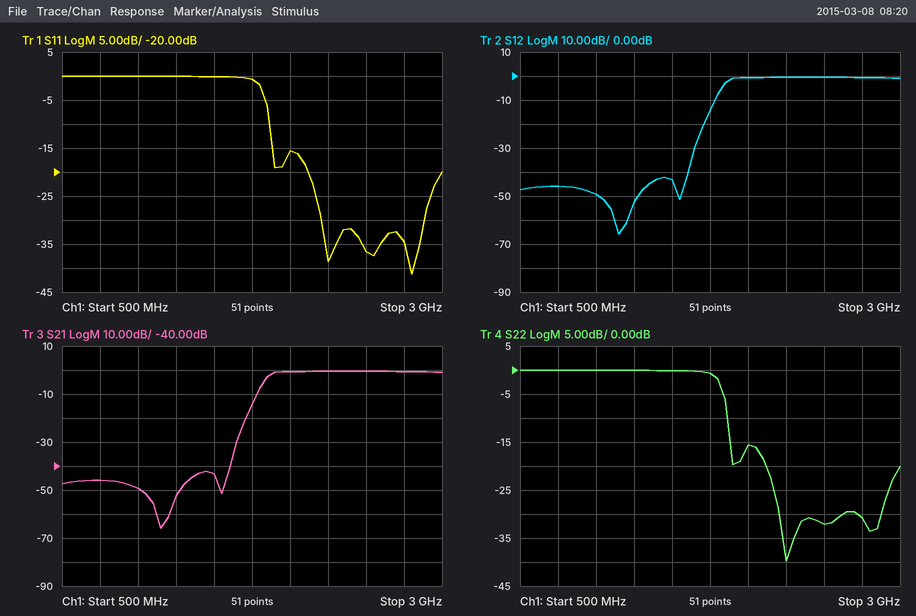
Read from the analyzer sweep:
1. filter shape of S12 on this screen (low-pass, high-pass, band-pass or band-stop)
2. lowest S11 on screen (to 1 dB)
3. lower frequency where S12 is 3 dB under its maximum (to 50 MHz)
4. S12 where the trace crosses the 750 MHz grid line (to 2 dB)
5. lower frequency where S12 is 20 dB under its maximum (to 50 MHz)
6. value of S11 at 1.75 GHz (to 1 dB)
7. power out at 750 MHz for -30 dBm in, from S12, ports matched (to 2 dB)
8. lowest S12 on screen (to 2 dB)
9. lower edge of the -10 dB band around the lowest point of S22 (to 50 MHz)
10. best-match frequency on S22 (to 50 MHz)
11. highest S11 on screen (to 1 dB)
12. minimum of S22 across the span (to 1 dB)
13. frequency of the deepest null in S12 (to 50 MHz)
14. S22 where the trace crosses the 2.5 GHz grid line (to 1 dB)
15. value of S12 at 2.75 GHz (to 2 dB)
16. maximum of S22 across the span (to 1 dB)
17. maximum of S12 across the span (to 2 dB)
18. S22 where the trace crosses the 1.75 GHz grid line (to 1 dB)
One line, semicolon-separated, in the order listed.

high-pass; -41 dB; 1.85 GHz; -46 dB; 1.70 GHz; -1 dB; -76 dBm; -66 dB; 1.85 GHz; 2.25 GHz; 0 dB; -40 dB; 1.15 GHz; -32 dB; 0 dB; 0 dB; 0 dB; -1 dB
